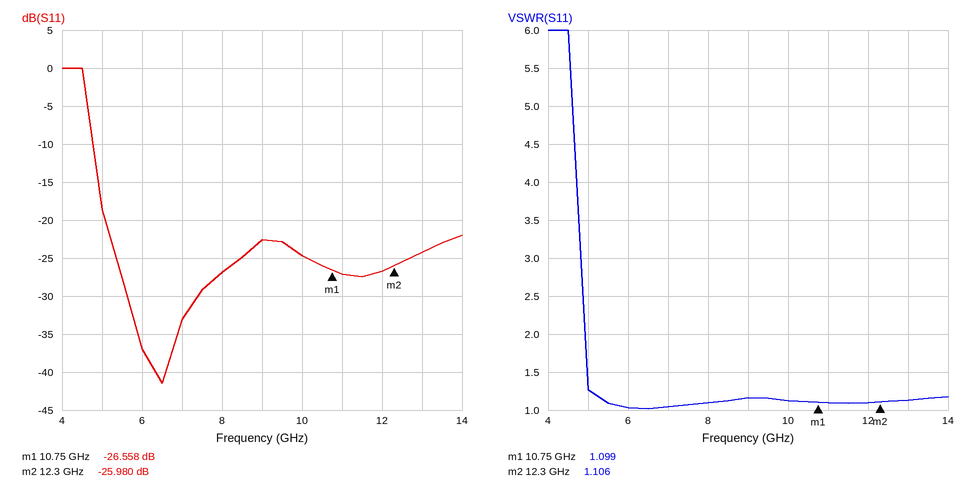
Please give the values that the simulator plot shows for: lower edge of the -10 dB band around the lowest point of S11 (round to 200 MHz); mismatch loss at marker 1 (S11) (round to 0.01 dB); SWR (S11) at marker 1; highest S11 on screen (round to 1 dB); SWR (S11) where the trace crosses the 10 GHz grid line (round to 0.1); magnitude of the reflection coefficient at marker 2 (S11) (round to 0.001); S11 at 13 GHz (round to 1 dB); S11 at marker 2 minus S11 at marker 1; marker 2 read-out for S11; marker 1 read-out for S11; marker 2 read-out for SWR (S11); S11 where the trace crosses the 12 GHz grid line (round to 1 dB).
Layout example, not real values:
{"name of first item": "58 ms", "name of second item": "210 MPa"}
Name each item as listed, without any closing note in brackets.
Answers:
{"lower edge of the -10 dB band around the lowest point of S11": "4.8 GHz", "mismatch loss at marker 1 (S11)": "0.01 dB", "SWR (S11) at marker 1": "1.099", "highest S11 on screen": "0 dB", "SWR (S11) where the trace crosses the 10 GHz grid line": "1.1", "magnitude of the reflection coefficient at marker 2 (S11)": "0.050", "S11 at 13 GHz": "-24 dB", "S11 at marker 2 minus S11 at marker 1": "0.578 dB", "marker 2 read-out for S11": "-25.980 dB", "marker 1 read-out for S11": "-26.558 dB", "marker 2 read-out for SWR": "1.106", "S11 where the trace crosses the 12 GHz grid line": "-27 dB"}
